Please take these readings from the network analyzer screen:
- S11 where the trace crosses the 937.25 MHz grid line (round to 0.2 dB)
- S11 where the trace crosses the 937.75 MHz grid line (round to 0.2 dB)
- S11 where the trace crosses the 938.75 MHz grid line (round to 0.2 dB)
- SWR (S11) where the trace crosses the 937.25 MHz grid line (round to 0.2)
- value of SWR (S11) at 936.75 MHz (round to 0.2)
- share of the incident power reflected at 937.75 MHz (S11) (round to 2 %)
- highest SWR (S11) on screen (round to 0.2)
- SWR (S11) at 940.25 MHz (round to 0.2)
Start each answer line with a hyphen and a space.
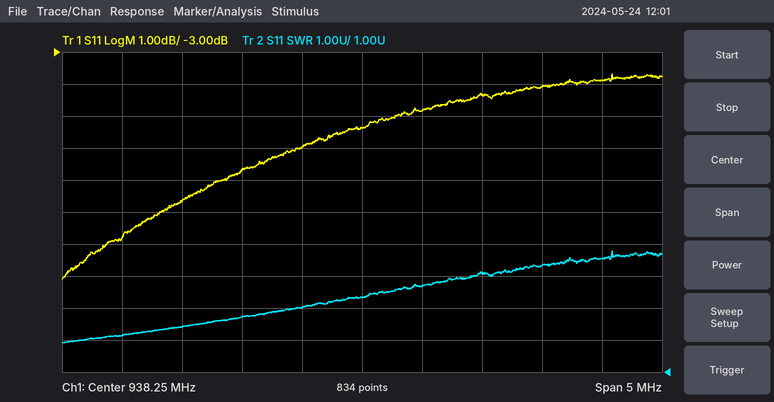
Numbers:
- -6.6 dB
- -6.0 dB
- -4.8 dB
- 2.8
- 2.4
- 26 %
- 4.8
- 4.6
